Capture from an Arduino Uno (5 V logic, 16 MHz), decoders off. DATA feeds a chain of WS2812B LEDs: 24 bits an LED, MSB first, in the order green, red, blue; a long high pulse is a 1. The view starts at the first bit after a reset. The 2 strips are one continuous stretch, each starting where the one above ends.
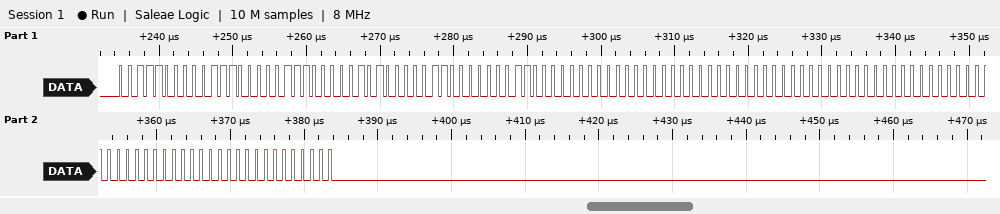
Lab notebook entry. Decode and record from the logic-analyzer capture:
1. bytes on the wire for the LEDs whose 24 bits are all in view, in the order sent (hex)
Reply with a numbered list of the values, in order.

1. 38 38 38 28 30 18 00 00 00 00 00 00 00 00 00
